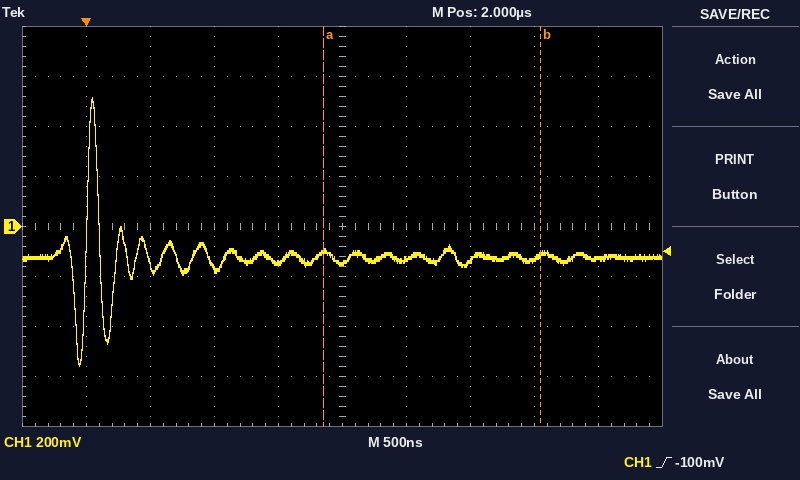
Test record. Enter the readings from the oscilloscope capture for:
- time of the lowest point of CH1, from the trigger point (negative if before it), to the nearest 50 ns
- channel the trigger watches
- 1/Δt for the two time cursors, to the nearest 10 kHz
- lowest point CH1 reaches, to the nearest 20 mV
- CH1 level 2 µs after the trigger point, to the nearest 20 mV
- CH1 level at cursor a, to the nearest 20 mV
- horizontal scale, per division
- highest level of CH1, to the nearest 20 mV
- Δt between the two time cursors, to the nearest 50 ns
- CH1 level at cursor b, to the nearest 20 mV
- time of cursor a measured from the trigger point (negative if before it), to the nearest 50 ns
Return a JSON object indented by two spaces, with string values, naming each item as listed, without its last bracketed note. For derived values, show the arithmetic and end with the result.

{
  "time of the lowest point of CH1, from the trigger point (negative if before it), to the nearest 50 ns": "-50 ns",
  "channel the trigger watches": "CH1",
  "1/Δt for the two time cursors, to the nearest 10 kHz": "1 / 1.70 µs ≈ 590 kHz",
  "lowest point CH1 reaches, to the nearest 20 mV": "-560 mV",
  "CH1 level 2 µs after the trigger point, to the nearest 20 mV": "-140 mV",
  "CH1 level at cursor a, to the nearest 20 mV": "-100 mV",
  "horizontal scale, per division": "500 ns",
  "highest level of CH1, to the nearest 20 mV": "520 mV",
  "Δt between the two time cursors, to the nearest 50 ns": "1.70 µs",
  "CH1 level at cursor b, to the nearest 20 mV": "-120 mV",
  "time of cursor a measured from the trigger point (negative if before it), to the nearest 50 ns": "+1.85 µs"
}
